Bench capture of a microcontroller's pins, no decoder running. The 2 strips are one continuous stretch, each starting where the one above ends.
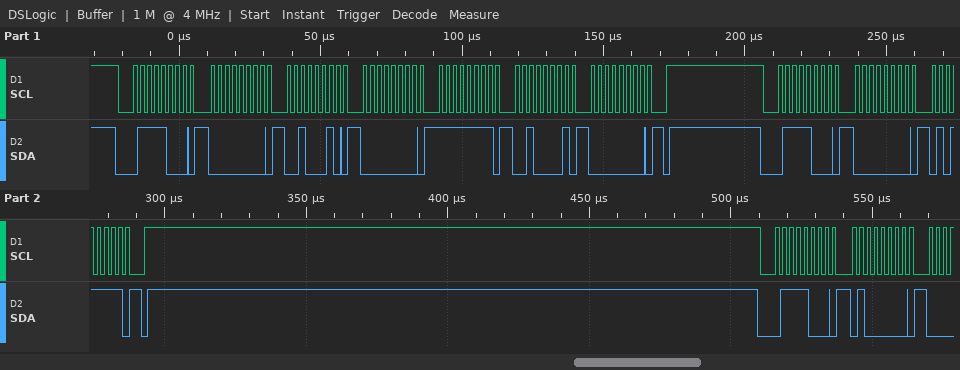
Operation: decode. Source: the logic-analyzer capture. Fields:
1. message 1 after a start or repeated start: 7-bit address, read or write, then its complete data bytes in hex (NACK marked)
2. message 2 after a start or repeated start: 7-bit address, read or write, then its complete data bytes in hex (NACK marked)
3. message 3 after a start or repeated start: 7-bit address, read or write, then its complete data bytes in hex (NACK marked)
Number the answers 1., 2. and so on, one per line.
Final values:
1. 0x3C write: 00 22 00 FF 21 00
2. 0x3C write: 00 5F
3. 0x3C write: 40
